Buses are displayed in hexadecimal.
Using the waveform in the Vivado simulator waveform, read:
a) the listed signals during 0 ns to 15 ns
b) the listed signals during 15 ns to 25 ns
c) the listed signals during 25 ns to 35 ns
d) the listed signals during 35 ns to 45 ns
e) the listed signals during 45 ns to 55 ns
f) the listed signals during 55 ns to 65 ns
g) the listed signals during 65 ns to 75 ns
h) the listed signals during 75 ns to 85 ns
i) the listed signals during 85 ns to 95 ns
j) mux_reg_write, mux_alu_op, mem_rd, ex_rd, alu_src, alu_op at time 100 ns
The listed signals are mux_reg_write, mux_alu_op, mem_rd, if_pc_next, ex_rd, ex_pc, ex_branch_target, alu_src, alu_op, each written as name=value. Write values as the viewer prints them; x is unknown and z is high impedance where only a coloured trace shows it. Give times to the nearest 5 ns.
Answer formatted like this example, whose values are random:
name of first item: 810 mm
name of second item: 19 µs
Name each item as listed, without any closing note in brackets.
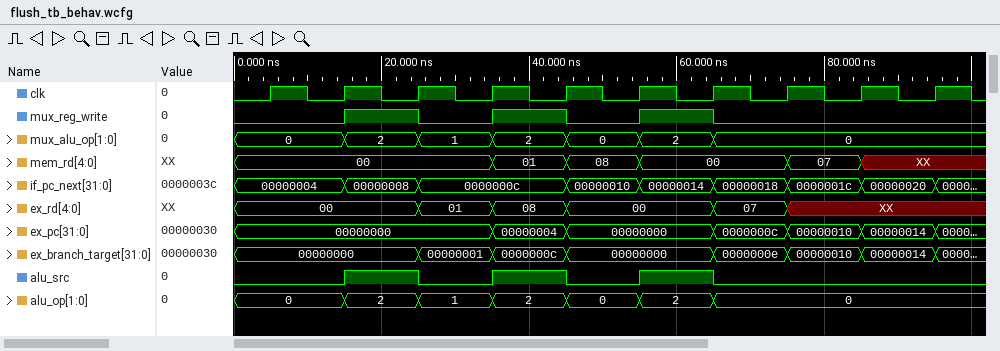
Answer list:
the listed signals during 0 ns to 15 ns: mux_reg_write=0, mux_alu_op=0, mem_rd=00, if_pc_next=00000004, ex_rd=00, ex_pc=00000000, ex_branch_target=00000000, alu_src=0, alu_op=0
the listed signals during 15 ns to 25 ns: mux_reg_write=1, mux_alu_op=2, mem_rd=00, if_pc_next=00000008, ex_rd=00, ex_pc=00000000, ex_branch_target=00000000, alu_src=1, alu_op=2
the listed signals during 25 ns to 35 ns: mux_reg_write=0, mux_alu_op=1, mem_rd=00, if_pc_next=0000000c, ex_rd=01, ex_pc=00000000, ex_branch_target=00000001, alu_src=0, alu_op=1
the listed signals during 35 ns to 45 ns: mux_reg_write=1, mux_alu_op=2, mem_rd=01, if_pc_next=0000000c, ex_rd=08, ex_pc=00000004, ex_branch_target=0000000c, alu_src=1, alu_op=2
the listed signals during 45 ns to 55 ns: mux_reg_write=0, mux_alu_op=0, mem_rd=08, if_pc_next=00000010, ex_rd=00, ex_pc=00000000, ex_branch_target=00000000, alu_src=0, alu_op=0
the listed signals during 55 ns to 65 ns: mux_reg_write=1, mux_alu_op=2, mem_rd=00, if_pc_next=00000014, ex_rd=00, ex_pc=00000000, ex_branch_target=00000000, alu_src=1, alu_op=2
the listed signals during 65 ns to 75 ns: mux_reg_write=0, mux_alu_op=0, mem_rd=00, if_pc_next=00000018, ex_rd=07, ex_pc=0000000c, ex_branch_target=0000000e, alu_src=0, alu_op=0
the listed signals during 75 ns to 85 ns: mux_reg_write=0, mux_alu_op=0, mem_rd=07, if_pc_next=0000001c, ex_rd=XX, ex_pc=00000010, ex_branch_target=00000010, alu_src=0, alu_op=0
the listed signals during 85 ns to 95 ns: mux_reg_write=0, mux_alu_op=0, mem_rd=XX, if_pc_next=00000020, ex_rd=XX, ex_pc=00000014, ex_branch_target=00000014, alu_src=0, alu_op=0
mux_reg_write, mux_alu_op, mem_rd, ex_rd, alu_src, alu_op at time 100 ns: mux_reg_write=0, mux_alu_op=0, mem_rd=XX, ex_rd=XX, alu_src=0, alu_op=0
